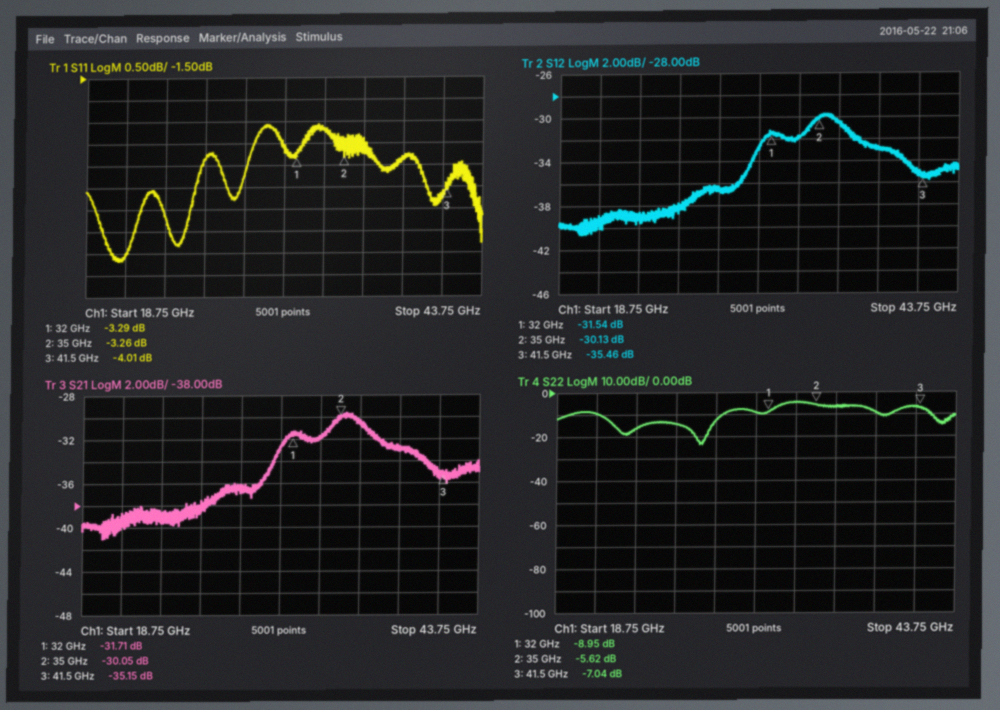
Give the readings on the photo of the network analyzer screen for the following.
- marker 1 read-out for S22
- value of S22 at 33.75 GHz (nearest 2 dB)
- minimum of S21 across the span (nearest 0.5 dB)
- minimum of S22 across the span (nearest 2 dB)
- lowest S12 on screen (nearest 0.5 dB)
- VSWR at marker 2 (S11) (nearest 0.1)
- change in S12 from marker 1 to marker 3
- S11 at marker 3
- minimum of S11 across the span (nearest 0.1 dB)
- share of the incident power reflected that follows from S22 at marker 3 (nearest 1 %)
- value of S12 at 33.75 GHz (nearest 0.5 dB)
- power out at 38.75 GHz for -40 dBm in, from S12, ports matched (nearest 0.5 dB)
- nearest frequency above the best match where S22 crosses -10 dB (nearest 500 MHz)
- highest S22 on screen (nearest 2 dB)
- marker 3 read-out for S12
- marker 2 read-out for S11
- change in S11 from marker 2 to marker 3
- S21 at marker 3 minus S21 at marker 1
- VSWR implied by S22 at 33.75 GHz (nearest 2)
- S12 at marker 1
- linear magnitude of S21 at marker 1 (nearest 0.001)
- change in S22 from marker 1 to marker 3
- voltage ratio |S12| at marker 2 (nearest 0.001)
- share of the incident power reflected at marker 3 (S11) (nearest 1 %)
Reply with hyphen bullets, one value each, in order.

- -8.95 dB
- -4 dB
- -41.0 dB
- -24 dB
- -40.5 dB
- 5.4
- -3.92 dB
- -4.01 dB
- -5.7 dB
- 20 %
- -32.0 dB
- -73.0 dBm
- 29.0 GHz
- -4 dB
- -35.46 dB
- -3.26 dB
- -0.75 dB
- -3.44 dB
- 4
- -31.54 dB
- 0.026
- 1.91 dB
- 0.031
- 40 %
